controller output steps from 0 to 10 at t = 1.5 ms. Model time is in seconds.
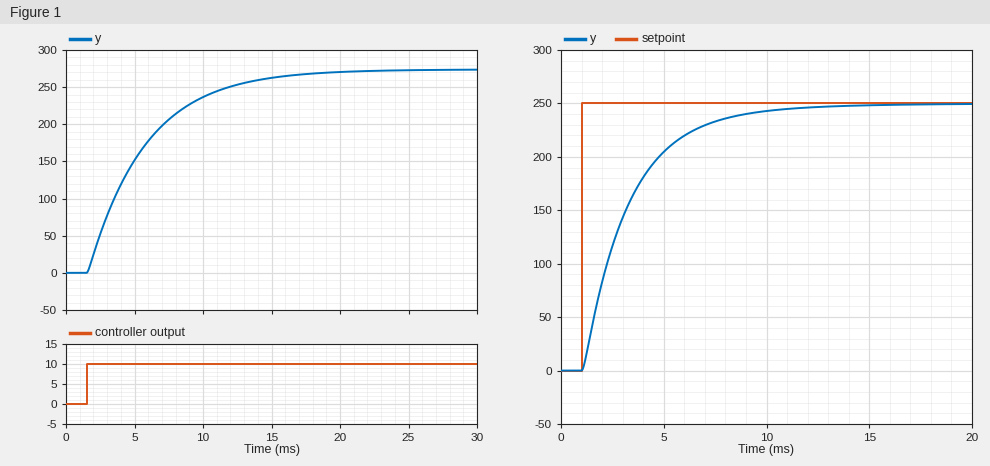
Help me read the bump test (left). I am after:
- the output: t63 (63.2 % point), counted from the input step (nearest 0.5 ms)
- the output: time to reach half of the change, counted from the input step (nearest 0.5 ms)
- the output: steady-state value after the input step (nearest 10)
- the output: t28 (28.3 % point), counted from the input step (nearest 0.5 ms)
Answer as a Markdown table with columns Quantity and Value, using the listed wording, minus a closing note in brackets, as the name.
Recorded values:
| Quantity | Value |
|---|---|
| the output: t63 (63.2 % point), counted from the input step | 4.5 ms |
| the output: time to reach half of the change, counted from the input step | 3.0 ms |
| the output: steady-state value after the input step | 270 |
| the output: t28 (28.3 % point), counted from the input step | 1.5 ms |
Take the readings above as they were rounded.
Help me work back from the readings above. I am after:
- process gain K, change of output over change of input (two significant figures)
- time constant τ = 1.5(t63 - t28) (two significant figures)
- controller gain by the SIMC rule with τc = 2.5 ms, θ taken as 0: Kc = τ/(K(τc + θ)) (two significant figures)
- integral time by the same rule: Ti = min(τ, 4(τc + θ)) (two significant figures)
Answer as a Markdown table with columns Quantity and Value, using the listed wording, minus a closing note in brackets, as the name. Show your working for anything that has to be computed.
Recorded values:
| Quantity | Value |
|---|---|
| process gain K, change of output over change of input | (270 - 0) / 10 = 27 |
| time constant τ = 1.5(t63 - t28) | 1.5 × (4.5 - 1.5) = 4.5 ms |
| controller gain by the SIMC rule with τc = 2.5 ms, θ taken as 0: Kc = τ/(K(τc + θ)) | 4.5 / (27 × (2.5 + 0)) = 0.067 |
| integral time by the same rule: Ti = min(τ, 4(τc + θ)) | min(4.5, 4 × (2.5 + 0)) = 4.5 ms |
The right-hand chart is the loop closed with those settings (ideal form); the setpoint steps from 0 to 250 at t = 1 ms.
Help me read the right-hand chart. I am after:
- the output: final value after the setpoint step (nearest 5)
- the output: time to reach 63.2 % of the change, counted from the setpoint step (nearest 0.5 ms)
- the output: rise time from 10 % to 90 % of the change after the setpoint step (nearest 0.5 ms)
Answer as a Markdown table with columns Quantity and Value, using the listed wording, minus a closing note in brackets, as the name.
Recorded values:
| Quantity | Value |
|---|---|
| the output: final value after the setpoint step | 250 |
| the output: time to reach 63.2 % of the change, counted from the setpoint step | 2.5 ms |
| the output: rise time from 10 % to 90 % of the change after the setpoint step | 5.0 ms |
